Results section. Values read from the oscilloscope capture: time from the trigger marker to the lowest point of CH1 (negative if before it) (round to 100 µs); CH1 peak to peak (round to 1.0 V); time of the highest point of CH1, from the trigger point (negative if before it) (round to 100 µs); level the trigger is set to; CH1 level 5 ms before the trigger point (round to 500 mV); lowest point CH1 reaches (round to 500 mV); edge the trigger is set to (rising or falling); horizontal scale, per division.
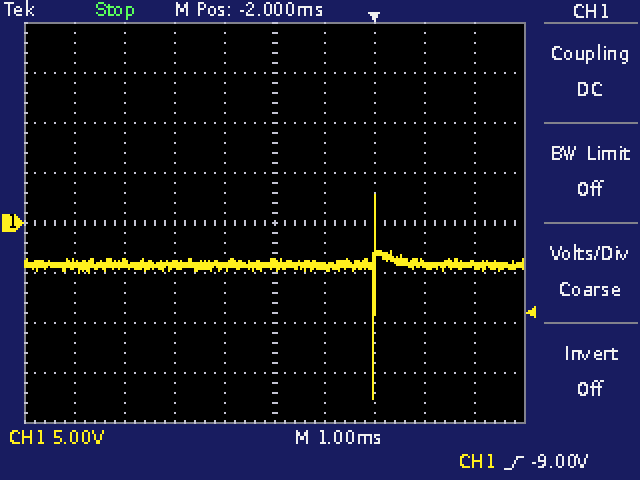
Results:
0.0 ms
20.0 V
0.0 ms
-9.00 V
-4.0 V
-17.5 V
rising
1 ms
